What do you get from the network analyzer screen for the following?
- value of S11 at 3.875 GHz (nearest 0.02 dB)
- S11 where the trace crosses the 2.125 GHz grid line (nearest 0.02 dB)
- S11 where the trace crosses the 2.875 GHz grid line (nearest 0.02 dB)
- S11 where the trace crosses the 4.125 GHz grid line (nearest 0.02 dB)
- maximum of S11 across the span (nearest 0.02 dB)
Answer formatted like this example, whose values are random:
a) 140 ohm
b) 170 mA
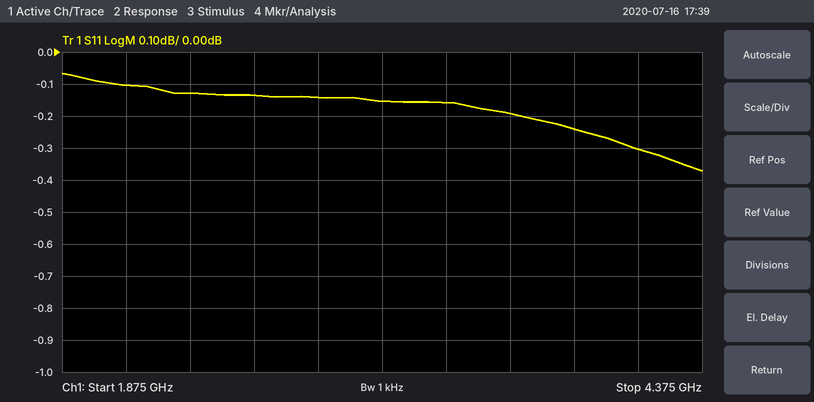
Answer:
a) -0.24 dB
b) -0.10 dB
c) -0.14 dB
d) -0.30 dB
e) -0.06 dB
